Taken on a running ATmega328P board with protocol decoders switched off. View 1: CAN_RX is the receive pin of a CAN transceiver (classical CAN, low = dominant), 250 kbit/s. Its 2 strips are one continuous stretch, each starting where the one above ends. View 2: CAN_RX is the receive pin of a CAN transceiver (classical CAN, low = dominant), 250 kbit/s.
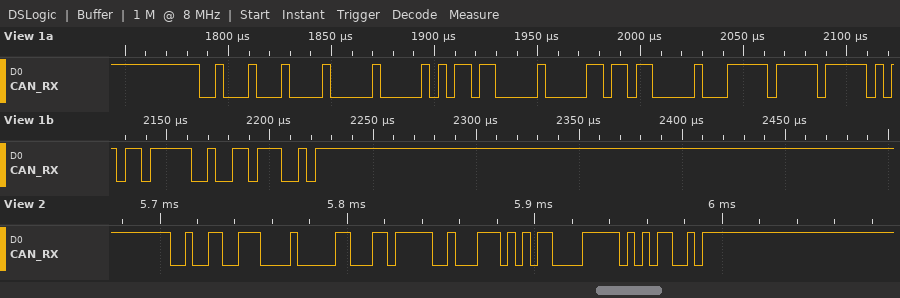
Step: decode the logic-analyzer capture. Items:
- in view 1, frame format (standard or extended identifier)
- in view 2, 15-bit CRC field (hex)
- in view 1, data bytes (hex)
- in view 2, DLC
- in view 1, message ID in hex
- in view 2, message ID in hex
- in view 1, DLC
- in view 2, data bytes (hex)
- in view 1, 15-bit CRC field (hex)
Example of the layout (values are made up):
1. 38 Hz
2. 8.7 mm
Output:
1. standard
2. 0x1FAC
3. 00 B6 00 5B 00 FF FF 5B
4. 4
5. 0x222
6. 0x267
7. 8
8. 11 BE 8E AC
9. 0x74DC
